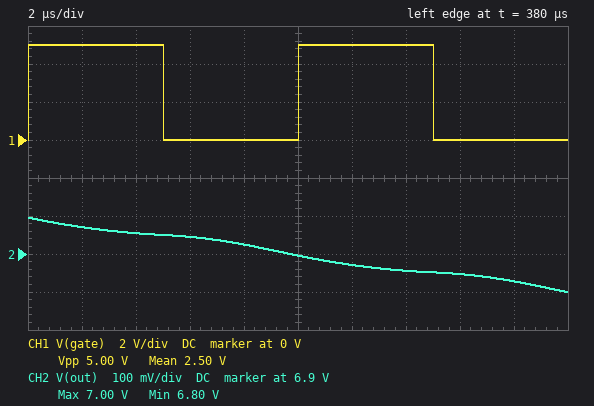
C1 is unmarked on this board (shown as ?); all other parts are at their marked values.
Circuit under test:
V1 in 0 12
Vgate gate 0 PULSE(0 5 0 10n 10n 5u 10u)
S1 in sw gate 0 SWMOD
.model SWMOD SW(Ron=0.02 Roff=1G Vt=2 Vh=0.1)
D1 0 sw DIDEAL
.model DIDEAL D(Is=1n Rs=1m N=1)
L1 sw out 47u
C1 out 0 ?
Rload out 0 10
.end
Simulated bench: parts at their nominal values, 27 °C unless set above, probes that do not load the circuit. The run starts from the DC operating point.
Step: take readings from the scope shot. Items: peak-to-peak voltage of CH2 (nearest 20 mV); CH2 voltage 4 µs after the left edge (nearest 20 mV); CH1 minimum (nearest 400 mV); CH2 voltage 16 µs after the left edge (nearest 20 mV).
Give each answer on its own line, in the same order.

200 mV
6.96 V
0 V
6.84 V
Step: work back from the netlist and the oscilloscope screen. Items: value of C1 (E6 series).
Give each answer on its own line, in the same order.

47 µF
